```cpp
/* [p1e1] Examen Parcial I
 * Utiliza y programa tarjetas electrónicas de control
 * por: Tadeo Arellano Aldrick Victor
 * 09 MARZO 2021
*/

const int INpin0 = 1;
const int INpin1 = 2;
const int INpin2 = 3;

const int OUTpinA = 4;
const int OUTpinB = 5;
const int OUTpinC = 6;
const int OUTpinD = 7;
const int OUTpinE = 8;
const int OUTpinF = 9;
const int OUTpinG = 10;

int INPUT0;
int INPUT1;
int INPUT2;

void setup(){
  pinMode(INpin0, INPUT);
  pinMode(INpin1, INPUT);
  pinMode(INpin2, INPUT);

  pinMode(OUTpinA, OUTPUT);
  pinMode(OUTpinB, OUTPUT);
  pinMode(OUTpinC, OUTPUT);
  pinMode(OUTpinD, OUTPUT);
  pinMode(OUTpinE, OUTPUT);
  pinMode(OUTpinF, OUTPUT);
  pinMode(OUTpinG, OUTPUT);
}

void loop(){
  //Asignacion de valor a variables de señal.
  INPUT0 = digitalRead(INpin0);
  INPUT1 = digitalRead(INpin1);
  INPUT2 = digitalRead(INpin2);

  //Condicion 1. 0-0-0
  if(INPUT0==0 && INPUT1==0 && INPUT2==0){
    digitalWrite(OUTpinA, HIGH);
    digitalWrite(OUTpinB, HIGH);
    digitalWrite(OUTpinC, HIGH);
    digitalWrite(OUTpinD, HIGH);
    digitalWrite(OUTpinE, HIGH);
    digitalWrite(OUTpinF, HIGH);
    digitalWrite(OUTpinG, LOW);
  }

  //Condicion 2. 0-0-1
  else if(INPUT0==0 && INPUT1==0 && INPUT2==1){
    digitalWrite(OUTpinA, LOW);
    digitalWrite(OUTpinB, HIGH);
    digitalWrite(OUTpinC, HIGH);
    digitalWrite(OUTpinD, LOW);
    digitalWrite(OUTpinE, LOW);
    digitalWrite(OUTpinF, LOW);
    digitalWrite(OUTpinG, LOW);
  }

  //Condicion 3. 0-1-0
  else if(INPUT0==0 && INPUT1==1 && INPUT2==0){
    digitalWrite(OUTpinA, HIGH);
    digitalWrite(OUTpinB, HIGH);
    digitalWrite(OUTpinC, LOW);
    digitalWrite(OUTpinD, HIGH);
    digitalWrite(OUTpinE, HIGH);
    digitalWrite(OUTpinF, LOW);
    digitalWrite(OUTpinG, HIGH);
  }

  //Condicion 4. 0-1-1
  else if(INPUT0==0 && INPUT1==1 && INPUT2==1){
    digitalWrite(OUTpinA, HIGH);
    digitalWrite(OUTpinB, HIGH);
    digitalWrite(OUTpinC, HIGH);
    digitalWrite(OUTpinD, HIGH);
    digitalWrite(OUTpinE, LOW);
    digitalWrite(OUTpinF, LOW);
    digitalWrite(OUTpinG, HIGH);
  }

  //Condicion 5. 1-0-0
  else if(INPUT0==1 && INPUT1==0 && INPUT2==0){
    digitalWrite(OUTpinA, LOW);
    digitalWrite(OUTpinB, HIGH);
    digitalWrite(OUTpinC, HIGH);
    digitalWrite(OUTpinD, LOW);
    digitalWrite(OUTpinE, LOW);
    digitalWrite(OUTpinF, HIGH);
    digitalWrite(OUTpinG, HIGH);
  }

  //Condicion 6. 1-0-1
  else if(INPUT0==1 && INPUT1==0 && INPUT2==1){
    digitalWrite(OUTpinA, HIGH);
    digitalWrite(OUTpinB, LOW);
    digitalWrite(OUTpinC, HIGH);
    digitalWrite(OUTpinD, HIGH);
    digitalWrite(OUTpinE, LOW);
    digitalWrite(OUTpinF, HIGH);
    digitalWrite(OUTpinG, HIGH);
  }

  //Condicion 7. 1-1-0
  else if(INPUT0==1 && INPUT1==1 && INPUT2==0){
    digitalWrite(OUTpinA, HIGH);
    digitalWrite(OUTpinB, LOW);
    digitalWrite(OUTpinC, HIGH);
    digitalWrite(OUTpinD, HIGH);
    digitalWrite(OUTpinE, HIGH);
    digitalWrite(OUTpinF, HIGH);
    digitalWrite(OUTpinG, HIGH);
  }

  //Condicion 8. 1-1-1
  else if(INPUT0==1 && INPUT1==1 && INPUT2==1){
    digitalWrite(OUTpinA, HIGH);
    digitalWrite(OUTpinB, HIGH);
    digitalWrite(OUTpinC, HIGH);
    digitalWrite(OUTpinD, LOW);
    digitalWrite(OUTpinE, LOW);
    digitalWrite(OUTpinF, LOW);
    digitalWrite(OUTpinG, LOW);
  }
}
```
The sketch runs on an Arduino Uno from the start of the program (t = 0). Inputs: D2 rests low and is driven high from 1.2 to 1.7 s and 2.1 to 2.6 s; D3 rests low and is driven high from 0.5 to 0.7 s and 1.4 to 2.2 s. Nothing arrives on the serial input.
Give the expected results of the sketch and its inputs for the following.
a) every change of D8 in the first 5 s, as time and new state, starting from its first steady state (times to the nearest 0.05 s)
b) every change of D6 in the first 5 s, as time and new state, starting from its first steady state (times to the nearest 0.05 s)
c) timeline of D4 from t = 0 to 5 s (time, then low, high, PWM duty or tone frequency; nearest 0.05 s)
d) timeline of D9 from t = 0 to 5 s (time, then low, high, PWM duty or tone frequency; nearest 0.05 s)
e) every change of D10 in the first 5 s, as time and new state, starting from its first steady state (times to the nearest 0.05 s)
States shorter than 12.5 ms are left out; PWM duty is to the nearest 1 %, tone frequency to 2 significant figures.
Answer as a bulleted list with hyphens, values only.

- 0 s high; 0.5 s low; 0.7 s high; 1.4 s low; 2.2 s high
- 0 s high; 1.2 s low; 1.4 s high; 2.2 s low; 2.6 s high
- 0 s high; 0.5 s low; 0.7 s high; 1.7 s low; 2.1 s high
- 0 s high; 0.5 s low; 0.7 s high; 1.2 s low; 2.6 s high
- 0 s low; 1.2 s high; 1.7 s low; 2.1 s high; 2.6 s low
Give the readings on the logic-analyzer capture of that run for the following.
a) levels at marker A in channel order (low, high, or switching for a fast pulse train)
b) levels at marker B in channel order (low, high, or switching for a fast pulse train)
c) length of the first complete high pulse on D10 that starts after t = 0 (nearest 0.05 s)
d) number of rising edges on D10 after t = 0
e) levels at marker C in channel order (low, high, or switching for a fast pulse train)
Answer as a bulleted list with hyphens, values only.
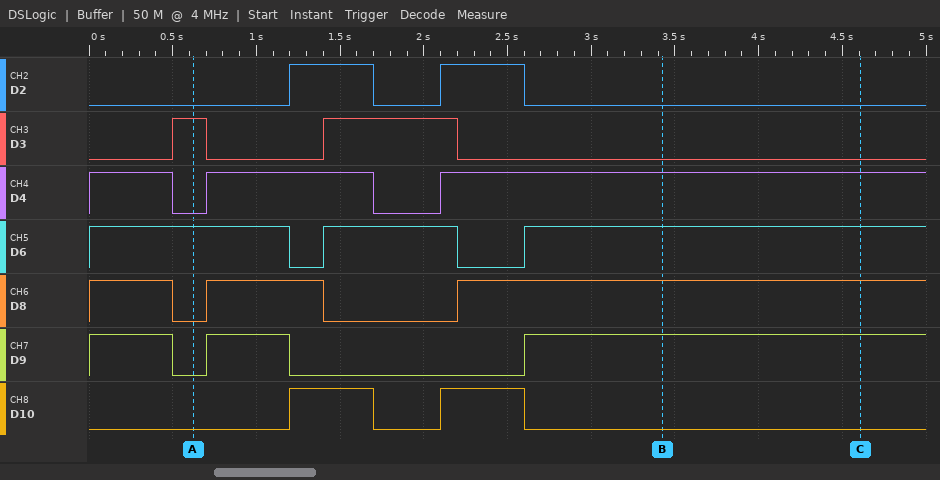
- D2 low, D3 high, D4 low, D6 high, D8 low, D9 low, D10 low
- D2 low, D3 low, D4 high, D6 high, D8 high, D9 high, D10 low
- 0.50 s
- 2
- D2 low, D3 low, D4 high, D6 high, D8 high, D9 high, D10 low
